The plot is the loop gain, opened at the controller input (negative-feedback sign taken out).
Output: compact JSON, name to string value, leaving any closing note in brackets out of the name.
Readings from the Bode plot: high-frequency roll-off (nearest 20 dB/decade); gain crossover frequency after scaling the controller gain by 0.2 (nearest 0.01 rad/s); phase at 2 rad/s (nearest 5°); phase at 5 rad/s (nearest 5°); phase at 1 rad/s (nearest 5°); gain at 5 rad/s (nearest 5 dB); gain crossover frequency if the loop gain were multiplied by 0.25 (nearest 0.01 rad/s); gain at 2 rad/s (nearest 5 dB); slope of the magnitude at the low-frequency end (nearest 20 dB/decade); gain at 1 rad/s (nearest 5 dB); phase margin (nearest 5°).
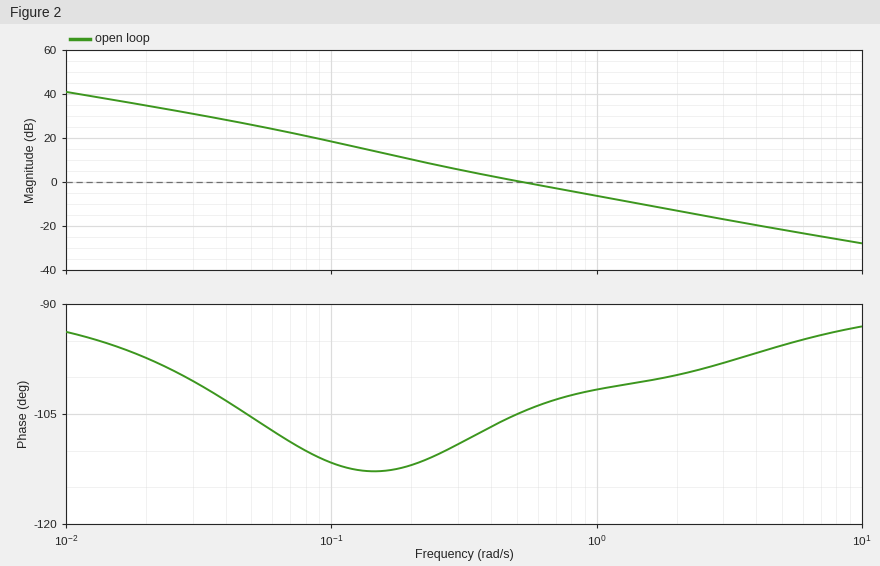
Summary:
{"high-frequency roll-off": "-20 dB/decade", "gain crossover frequency after scaling the controller gain by 0.2": "0.15 rad/s", "phase at 2 rad/s": "-100°", "phase at 5 rad/s": "-95°", "phase at 1 rad/s": "-100°", "gain at 5 rad/s": "-20 dB", "gain crossover frequency if the loop gain were multiplied by 0.25": "0.17 rad/s", "gain at 2 rad/s": "-15 dB", "slope of the magnitude at the low-frequency end": "-20 dB/decade", "gain at 1 rad/s": "-5 dB", "phase margin": "75°"}
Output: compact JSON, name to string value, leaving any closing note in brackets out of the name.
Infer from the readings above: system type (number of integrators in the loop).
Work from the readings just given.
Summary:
{"system type": "1"}
